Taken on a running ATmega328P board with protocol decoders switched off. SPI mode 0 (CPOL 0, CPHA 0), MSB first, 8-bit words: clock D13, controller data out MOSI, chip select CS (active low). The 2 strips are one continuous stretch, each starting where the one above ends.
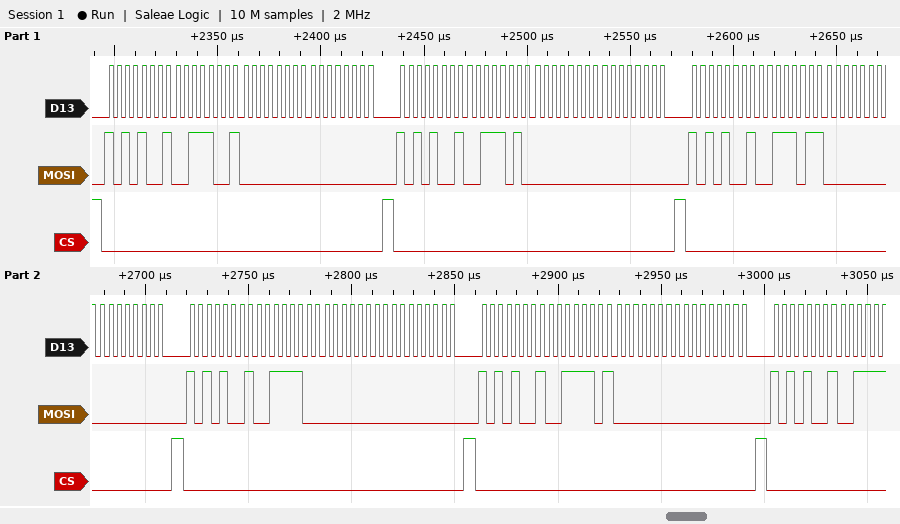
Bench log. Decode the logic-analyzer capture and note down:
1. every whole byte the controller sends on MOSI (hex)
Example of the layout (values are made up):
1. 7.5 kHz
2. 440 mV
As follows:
1. A9 39 00 00 A9 3A 00 00 A9 3B 00 00 A9 3C 00 00 A9 3D 00 00 A9
